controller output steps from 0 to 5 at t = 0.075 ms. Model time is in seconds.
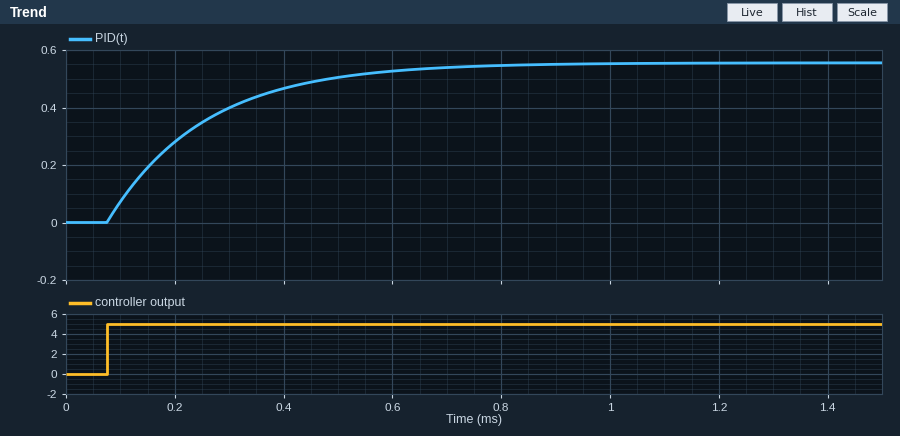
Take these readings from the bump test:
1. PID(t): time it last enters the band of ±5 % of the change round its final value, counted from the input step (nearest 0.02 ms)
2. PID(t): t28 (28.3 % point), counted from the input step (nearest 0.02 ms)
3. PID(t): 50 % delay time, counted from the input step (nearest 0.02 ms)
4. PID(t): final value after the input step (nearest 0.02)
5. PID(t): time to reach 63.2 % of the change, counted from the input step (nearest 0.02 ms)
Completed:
0.54 ms
0.06 ms
0.12 ms
0.56
0.18 ms
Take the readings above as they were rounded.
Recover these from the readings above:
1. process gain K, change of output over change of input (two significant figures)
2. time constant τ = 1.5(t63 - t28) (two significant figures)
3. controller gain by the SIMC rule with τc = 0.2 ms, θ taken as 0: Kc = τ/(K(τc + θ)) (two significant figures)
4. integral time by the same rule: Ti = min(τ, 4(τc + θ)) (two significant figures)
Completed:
0.11
0.18 ms
8.2
0.18 ms
